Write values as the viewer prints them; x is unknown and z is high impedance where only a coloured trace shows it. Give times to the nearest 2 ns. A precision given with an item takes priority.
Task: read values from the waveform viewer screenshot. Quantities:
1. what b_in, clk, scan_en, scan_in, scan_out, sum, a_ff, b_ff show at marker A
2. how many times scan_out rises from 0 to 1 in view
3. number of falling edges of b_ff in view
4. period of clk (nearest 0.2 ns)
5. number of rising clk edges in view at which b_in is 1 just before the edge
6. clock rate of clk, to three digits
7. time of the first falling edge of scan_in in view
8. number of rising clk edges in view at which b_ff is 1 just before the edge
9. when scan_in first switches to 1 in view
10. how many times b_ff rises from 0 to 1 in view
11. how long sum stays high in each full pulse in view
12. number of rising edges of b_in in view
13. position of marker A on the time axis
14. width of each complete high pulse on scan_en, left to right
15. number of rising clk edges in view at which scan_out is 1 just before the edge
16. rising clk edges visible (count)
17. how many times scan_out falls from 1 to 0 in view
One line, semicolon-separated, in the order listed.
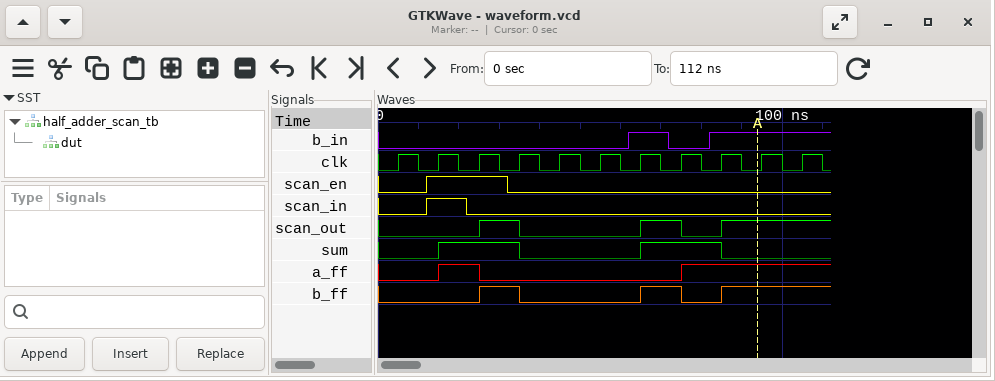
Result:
b_in=1, clk=0, scan_en=0, scan_in=0, scan_out=1, sum=0, a_ff=1, b_ff=1; 3; 2; 10 ns; 4; 100 MHz; 22 ns; 4; 12 ns; 3; 20 ns, 20 ns; 2; 94 ns; 20 ns; 4; 11; 2
